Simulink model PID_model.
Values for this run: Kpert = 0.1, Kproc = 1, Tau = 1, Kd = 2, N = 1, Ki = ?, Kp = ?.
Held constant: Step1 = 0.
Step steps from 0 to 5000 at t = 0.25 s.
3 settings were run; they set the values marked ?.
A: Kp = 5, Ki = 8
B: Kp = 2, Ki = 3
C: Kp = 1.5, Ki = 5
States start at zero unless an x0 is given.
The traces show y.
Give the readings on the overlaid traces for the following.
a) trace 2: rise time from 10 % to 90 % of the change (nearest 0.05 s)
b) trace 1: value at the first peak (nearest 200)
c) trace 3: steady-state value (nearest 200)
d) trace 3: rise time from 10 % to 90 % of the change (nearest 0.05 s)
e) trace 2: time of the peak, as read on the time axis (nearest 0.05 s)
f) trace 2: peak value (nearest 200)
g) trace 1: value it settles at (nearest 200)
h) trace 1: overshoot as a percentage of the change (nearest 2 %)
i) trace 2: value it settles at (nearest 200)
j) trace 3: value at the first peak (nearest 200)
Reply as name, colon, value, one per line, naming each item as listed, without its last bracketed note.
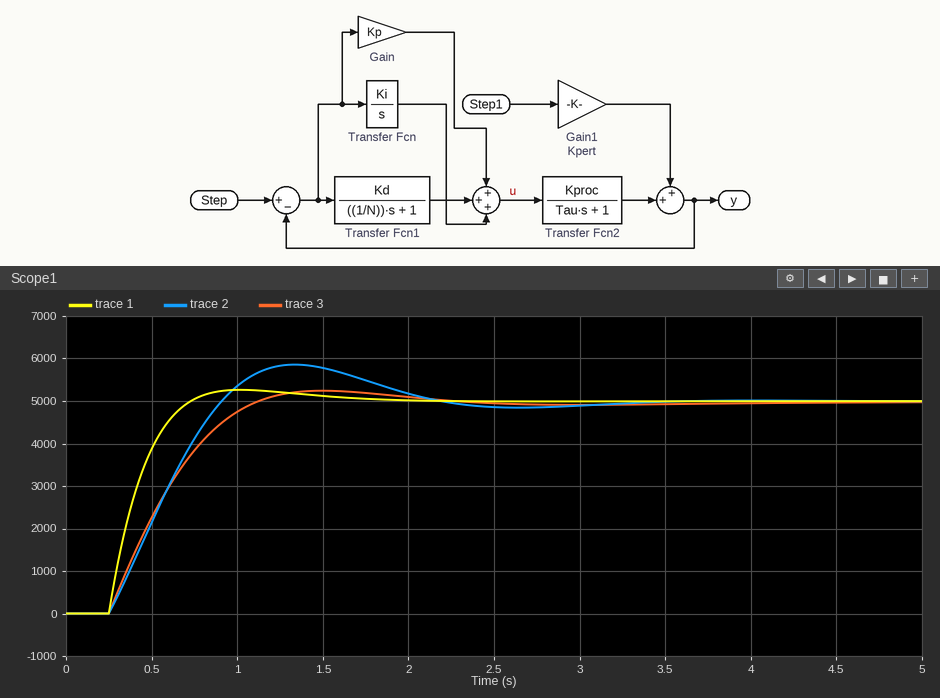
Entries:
trace 2: rise time from 10 % to 90 % of the change: 0.50 s
trace 1: value at the first peak: 5200
trace 3: steady-state value: 5000
trace 3: rise time from 10 % to 90 % of the change: 0.60 s
trace 2: time of the peak, as read on the time axis: 1.35 s
trace 2: peak value: 5800
trace 1: value it settles at: 5000
trace 1: overshoot as a percentage of the change: 6 %
trace 2: value it settles at: 5000
trace 3: value at the first peak: 5200
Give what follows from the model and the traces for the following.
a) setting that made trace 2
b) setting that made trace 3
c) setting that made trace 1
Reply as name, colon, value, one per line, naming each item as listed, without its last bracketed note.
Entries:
setting that made trace 2: C
setting that made trace 3: B
setting that made trace 1: A
